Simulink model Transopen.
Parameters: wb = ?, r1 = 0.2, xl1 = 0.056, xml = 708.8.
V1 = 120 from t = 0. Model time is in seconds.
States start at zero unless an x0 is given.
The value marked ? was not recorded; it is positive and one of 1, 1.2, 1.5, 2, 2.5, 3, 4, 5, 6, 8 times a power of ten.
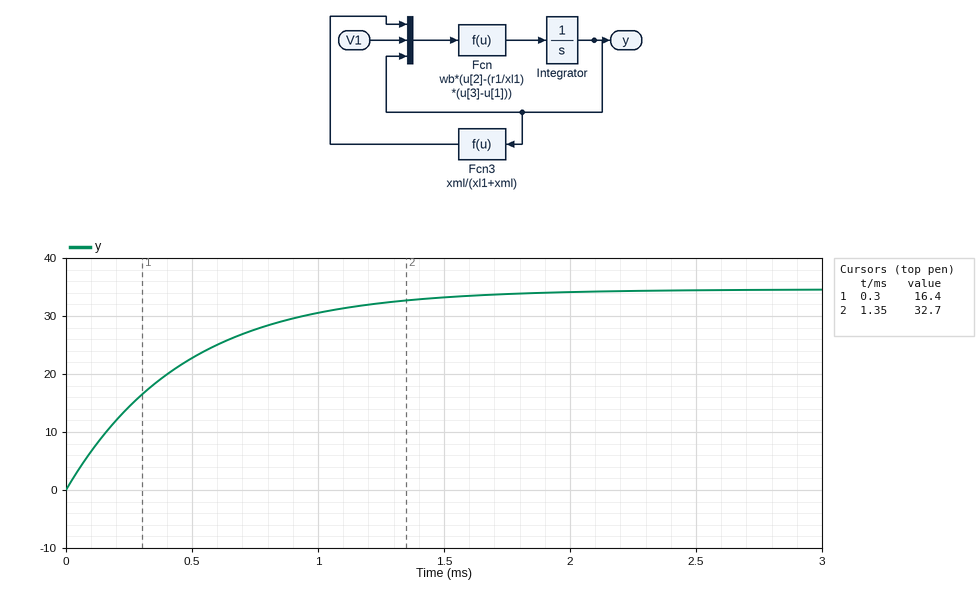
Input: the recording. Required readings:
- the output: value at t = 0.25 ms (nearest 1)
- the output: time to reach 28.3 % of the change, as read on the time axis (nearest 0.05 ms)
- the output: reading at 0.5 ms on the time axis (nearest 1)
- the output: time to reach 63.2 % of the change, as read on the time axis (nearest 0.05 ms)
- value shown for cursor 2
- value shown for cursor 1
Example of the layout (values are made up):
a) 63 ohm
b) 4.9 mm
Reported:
a) 14
b) 0.15 ms
c) 23
d) 0.45 ms
e) 32.7
f) 16.4
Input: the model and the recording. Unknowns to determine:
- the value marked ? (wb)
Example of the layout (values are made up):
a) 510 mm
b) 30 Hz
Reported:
a) 600
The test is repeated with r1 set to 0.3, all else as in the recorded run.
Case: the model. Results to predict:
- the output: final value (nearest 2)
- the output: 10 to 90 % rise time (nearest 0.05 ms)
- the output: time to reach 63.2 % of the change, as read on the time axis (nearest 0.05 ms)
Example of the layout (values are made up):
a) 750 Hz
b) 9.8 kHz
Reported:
a) 24
b) 0.70 ms
c) 0.30 ms
